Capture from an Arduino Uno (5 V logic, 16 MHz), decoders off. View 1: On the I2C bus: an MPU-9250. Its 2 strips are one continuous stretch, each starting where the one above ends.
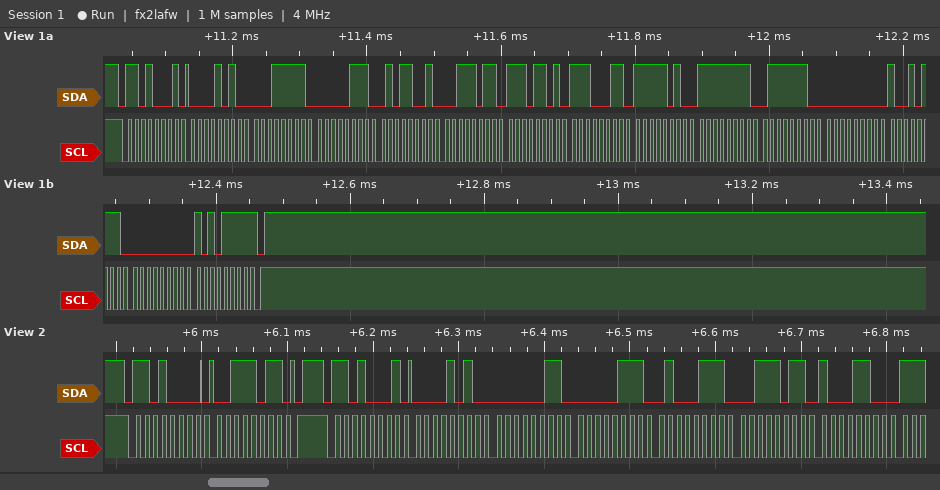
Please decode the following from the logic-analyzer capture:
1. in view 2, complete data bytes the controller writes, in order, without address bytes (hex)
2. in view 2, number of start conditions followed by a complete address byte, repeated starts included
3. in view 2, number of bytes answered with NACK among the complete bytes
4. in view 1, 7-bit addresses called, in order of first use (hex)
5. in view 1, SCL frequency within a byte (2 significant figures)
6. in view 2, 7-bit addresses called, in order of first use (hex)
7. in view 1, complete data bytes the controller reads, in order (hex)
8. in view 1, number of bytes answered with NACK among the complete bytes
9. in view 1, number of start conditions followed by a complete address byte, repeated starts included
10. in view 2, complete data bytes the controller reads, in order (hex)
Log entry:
3B
2
0
0x68
100 kHz
0x68
0A 1F 07 59 3B ED E3 FA FF 7E 00 97 00 AF
1
1
0A 03 07 47 3B 8C
